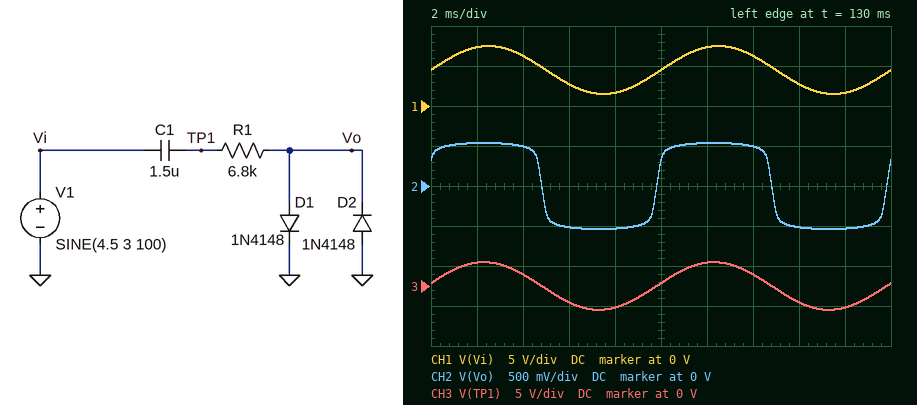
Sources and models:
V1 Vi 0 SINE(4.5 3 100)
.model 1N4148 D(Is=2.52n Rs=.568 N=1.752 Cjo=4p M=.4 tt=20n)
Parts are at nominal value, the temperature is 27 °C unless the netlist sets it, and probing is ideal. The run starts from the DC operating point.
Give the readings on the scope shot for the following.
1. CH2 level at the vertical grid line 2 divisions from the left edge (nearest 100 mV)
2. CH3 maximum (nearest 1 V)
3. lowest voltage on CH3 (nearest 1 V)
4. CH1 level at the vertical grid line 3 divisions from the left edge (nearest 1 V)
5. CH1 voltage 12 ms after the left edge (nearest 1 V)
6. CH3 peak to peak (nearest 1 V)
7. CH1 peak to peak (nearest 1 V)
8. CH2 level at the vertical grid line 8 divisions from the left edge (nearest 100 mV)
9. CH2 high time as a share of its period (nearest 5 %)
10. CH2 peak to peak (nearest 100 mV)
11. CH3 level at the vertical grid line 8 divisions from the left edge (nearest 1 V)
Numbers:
500 mV
3 V
-3 V
3 V
7 V
6 V
6 V
-500 mV
50 %
1.1 V
-2 V
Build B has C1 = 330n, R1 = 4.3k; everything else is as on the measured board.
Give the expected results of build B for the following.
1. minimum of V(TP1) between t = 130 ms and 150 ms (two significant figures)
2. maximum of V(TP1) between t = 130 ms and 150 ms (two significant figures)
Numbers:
-2.3 V
2.3 V
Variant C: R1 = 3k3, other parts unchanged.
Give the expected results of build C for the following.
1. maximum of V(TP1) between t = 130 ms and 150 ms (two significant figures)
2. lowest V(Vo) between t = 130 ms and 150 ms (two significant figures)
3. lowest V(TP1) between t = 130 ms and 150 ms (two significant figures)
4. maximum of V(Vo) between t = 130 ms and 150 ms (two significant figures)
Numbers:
2.9 V
-570 mV
-2.9 V
570 mV
